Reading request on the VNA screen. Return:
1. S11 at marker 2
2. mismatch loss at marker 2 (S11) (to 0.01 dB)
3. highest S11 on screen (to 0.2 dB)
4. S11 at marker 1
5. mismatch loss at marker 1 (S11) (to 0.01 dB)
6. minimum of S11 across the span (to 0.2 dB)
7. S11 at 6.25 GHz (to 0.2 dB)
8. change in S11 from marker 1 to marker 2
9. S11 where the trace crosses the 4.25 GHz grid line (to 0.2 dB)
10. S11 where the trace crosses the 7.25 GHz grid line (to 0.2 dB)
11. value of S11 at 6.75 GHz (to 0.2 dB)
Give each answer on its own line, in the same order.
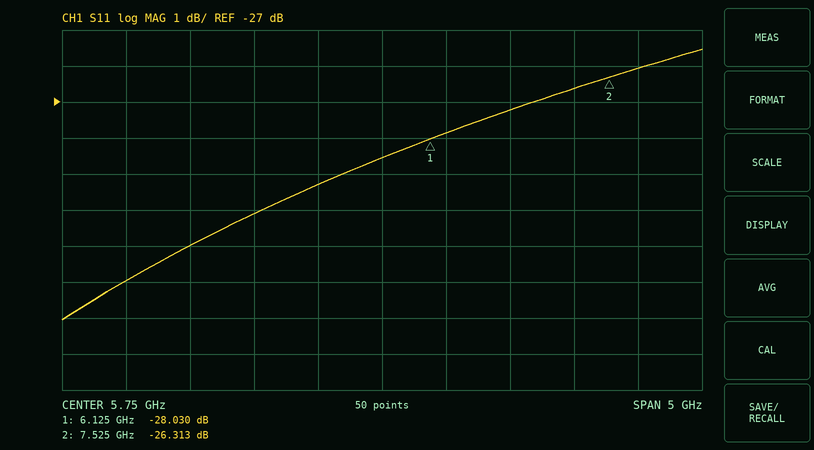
-26.313 dB
0.01 dB
-25.6 dB
-28.030 dB
0.01 dB
-33.0 dB
-27.8 dB
1.717 dB
-31.0 dB
-26.6 dB
-27.2 dB
